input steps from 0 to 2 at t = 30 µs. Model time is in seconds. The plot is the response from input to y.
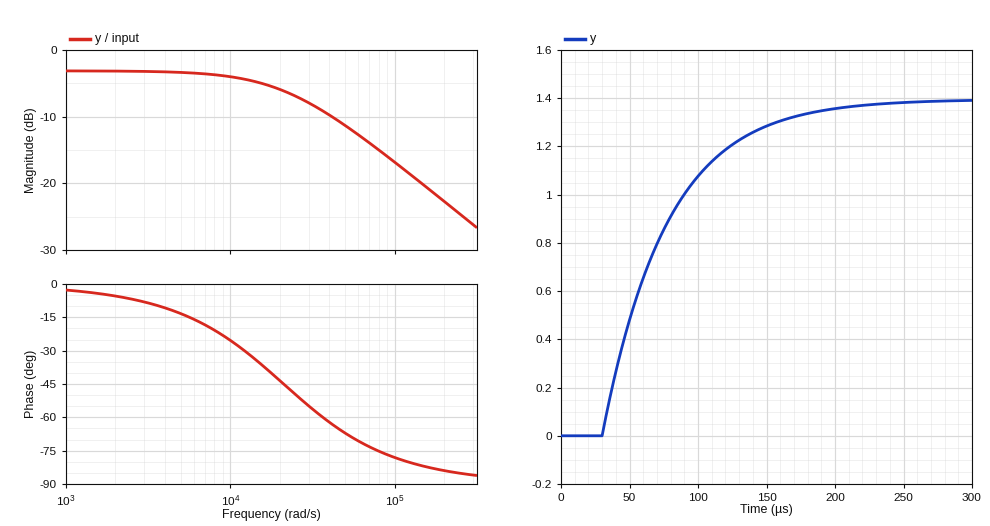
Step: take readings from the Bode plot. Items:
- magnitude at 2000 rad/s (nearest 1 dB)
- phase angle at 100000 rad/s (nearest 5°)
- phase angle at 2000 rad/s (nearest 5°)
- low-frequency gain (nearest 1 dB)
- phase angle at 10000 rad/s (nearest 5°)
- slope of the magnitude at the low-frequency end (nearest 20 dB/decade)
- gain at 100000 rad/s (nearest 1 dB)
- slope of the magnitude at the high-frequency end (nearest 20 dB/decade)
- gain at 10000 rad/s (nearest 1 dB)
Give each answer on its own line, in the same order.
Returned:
-3 dB
-80°
-5°
-3 dB
-25°
0 dB/decade
-17 dB
-20 dB/decade
-4 dB
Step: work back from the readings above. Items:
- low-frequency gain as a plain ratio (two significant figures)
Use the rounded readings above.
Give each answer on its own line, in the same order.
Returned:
0.71
